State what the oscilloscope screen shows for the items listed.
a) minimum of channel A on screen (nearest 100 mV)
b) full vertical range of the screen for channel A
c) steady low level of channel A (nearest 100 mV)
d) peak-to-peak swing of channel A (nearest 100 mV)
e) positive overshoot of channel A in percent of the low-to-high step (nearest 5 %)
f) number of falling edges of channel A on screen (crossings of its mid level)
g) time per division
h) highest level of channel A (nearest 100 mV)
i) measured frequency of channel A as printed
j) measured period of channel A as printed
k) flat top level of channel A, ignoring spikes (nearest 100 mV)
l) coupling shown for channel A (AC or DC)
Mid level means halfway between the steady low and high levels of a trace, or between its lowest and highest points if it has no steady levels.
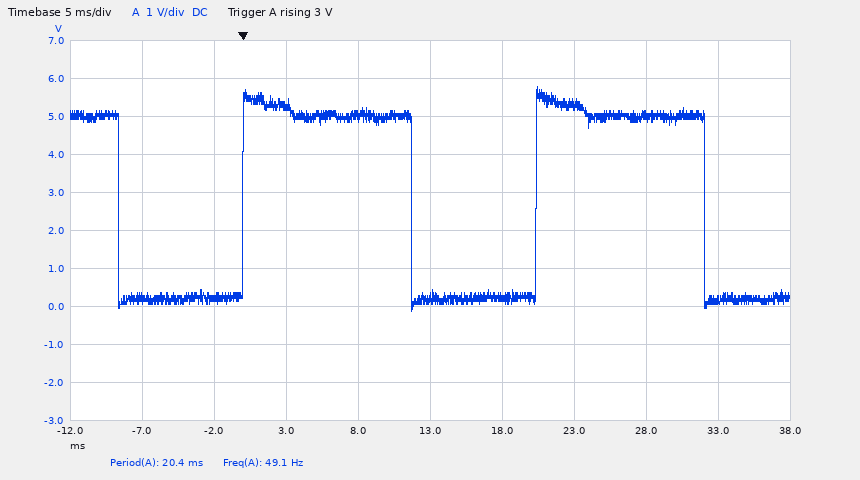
-100 mV
10 V
200 mV
5.9 V
15 %
3
5 ms
5.8 V
49.1 Hz
20.4 ms
5.0 V
DC
